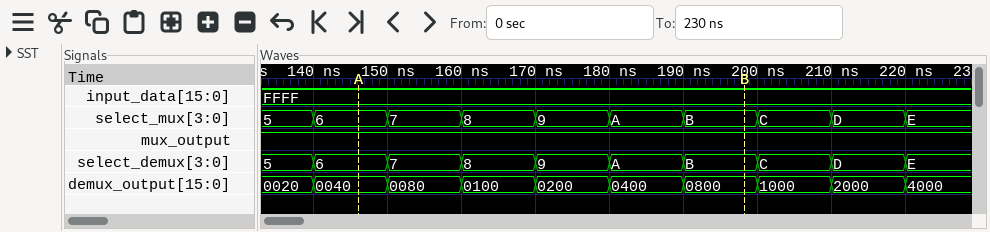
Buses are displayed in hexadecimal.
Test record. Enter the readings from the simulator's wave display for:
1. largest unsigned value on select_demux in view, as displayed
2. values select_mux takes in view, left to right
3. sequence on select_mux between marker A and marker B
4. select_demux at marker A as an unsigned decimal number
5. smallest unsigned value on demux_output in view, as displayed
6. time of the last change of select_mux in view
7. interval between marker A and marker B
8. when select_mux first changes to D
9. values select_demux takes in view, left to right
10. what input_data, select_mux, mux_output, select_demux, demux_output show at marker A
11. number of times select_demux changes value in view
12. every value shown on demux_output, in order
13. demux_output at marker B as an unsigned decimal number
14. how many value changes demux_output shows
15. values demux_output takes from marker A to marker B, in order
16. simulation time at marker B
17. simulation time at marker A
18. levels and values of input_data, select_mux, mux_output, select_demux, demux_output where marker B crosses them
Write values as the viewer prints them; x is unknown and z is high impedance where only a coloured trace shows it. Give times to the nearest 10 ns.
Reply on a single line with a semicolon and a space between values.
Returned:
E; 5, 6, 7, 8, 9, A, B, C, D, E; 6, 7, 8, 9, A, B; 6; 0020; 220 ns; 50 ns; 210 ns; 5, 6, 7, 8, 9, A, B, C, D, E; input_data=FFFF, select_mux=6, mux_output=1, select_demux=6, demux_output=0040; 9; 0020, 0040, 0080, 0100, 0200, 0400, 0800, 1000, 2000, 4000; 2048; 9; 0040, 0080, 0100, 0200, 0400, 0800; 200 ns; 150 ns; input_data=FFFF, select_mux=B, mux_output=1, select_demux=B, demux_output=0800
